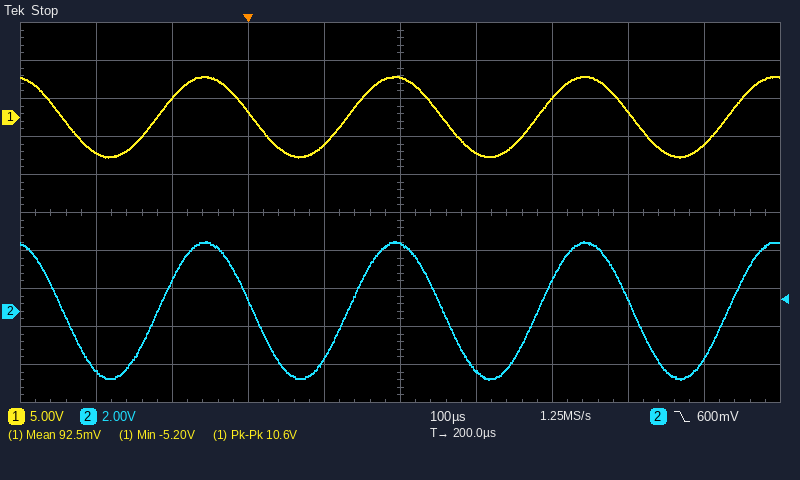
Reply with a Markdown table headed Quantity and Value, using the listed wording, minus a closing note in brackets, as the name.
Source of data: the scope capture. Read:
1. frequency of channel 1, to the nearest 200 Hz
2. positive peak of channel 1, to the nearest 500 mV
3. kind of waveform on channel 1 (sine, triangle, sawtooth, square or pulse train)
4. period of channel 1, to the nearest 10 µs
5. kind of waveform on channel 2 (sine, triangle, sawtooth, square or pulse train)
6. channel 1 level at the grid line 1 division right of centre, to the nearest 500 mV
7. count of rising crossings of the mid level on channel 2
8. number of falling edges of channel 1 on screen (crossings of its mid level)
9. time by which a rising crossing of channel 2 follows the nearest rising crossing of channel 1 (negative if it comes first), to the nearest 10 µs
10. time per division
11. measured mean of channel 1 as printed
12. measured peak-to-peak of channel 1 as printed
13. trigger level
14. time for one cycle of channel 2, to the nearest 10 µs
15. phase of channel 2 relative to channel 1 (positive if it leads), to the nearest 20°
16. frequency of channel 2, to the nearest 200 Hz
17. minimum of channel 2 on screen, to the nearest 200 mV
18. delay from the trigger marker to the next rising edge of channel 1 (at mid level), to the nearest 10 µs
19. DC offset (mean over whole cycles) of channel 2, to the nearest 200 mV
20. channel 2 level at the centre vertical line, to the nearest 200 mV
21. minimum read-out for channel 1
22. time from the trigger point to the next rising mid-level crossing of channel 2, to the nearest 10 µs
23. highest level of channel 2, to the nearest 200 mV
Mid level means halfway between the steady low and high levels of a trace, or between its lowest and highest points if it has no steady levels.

| Quantity | Value |
|---|---|
| frequency of channel 1, to the nearest 200 Hz | 4.0 kHz |
| positive peak of channel 1, to the nearest 500 mV | 5.5 V |
| kind of waveform on channel 1 | sine |
| period of channel 1, to the nearest 10 µs | 250 µs |
| kind of waveform on channel 2 | sine |
| channel 1 level at the grid line 1 division right of centre, to the nearest 500 mV | -4.5 V |
| count of rising crossings of the mid level on channel 2 | 4 |
| number of falling edges of channel 1 on screen | 4 |
| time by which a rising crossing of channel 2 follows the nearest rising crossing of channel 1 (negative if it comes first), to the nearest 10 µs | 0 µs |
| time per division | 100 µs |
| measured mean of channel 1 as printed | 92.5 mV |
| measured peak-to-peak of channel 1 as printed | 10.6 V |
| trigger level | 600 mV |
| time for one cycle of channel 2, to the nearest 10 µs | 250 µs |
| phase of channel 2 relative to channel 1 (positive if it leads), to the nearest 20° | 0° |
| frequency of channel 2, to the nearest 200 Hz | 4.0 kHz |
| minimum of channel 2 on screen, to the nearest 200 mV | -3.6 V |
| delay from the trigger marker to the next rising edge of channel 1 (at mid level), to the nearest 10 µs | 130 µs |
| DC offset (mean over whole cycles) of channel 2, to the nearest 200 mV | 0.0 V |
| channel 2 level at the centre vertical line, to the nearest 200 mV | 3.6 V |
| minimum read-out for channel 1 | -5.20 V |
| time from the trigger point to the next rising mid-level crossing of channel 2, to the nearest 10 µs | 130 µs |
| highest level of channel 2, to the nearest 200 mV | 3.6 V |
